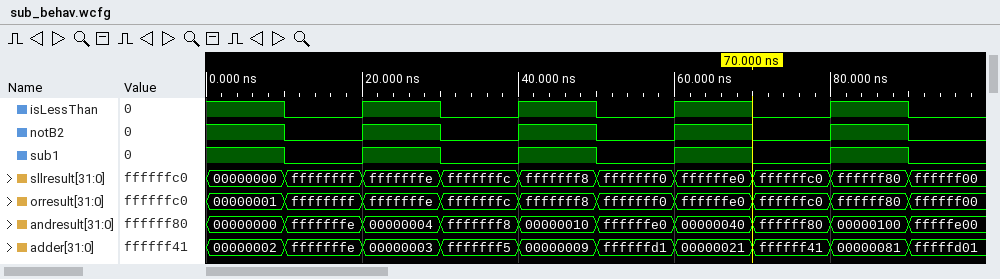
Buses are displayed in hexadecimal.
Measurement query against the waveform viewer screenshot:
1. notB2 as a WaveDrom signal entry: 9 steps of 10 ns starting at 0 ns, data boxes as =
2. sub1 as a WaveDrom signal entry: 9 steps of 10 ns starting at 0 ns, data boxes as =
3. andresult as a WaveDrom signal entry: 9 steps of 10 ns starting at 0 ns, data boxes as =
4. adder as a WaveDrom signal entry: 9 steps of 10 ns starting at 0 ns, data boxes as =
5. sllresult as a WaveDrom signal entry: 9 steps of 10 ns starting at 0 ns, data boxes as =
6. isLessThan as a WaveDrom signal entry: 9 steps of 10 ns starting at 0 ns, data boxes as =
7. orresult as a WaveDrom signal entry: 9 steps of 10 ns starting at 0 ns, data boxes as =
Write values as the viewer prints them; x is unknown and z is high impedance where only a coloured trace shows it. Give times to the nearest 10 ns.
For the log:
{name: 'notB2', wave: '101010101'}
{name: 'sub1', wave: '101010101'}
{name: 'andresult', wave: '=========', data: '00000000 fffffffe 00000004 fffffff8 00000010 ffffffe0 00000040 ffffff80 00000100'}
{name: 'adder', wave: '=========', data: '00000002 fffffffe 00000003 fffffff5 00000009 ffffffd1 00000021 ffffff41 00000081'}
{name: 'sllresult', wave: '=========', data: '00000000 ffffffff fffffffe fffffffc fffffff8 fffffff0 ffffffe0 ffffffc0 ffffff80'}
{name: 'isLessThan', wave: '101010101'}
{name: 'orresult', wave: '=========', data: '00000001 ffffffff fffffffe fffffffc fffffff8 fffffff0 ffffffe0 ffffffc0 ffffff80'}
